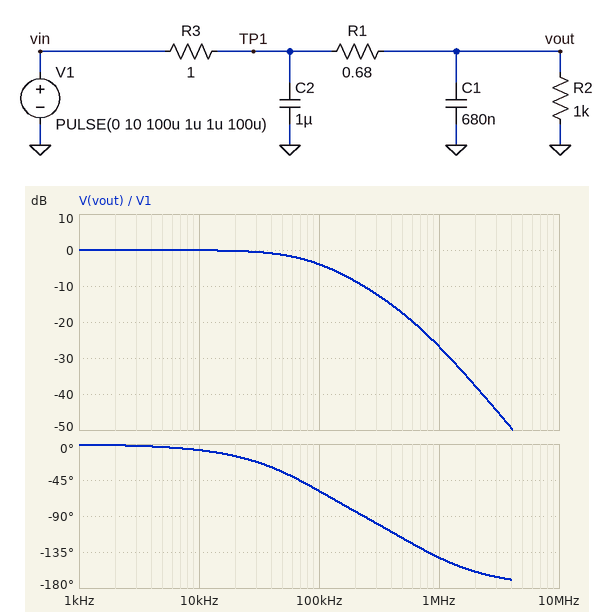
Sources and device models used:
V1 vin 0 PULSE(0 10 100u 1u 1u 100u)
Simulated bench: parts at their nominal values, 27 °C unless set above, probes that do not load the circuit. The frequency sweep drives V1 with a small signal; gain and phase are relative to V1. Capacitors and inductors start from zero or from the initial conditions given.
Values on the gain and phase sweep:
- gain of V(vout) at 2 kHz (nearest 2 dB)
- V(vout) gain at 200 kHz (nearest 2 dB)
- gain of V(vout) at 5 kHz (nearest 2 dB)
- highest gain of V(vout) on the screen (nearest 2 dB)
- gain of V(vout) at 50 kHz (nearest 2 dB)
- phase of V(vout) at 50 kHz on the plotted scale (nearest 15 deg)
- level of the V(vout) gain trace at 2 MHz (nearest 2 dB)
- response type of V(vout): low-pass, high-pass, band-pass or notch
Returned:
0 dB
-8 dB
0 dB
0 dB
-2 dB
-30 deg
-38 dB
low-pass
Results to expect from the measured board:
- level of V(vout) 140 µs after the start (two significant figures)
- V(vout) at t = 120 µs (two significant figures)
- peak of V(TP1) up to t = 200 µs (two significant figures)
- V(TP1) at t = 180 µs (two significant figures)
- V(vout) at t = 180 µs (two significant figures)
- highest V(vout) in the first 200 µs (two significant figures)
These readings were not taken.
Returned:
10 V
10 V
10 V
10 V
10 V
10 V
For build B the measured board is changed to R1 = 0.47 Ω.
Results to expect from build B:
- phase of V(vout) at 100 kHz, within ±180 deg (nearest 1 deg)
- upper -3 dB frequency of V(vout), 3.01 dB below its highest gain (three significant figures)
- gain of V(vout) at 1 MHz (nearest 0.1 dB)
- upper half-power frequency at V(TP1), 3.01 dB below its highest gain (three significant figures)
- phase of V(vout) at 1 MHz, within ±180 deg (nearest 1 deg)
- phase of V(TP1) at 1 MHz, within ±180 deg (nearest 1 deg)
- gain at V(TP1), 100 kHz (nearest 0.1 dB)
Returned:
-55 deg
86.6 kHz
-24.7 dB
89.3 kHz
-133 deg
-69 deg
-3.5 dB
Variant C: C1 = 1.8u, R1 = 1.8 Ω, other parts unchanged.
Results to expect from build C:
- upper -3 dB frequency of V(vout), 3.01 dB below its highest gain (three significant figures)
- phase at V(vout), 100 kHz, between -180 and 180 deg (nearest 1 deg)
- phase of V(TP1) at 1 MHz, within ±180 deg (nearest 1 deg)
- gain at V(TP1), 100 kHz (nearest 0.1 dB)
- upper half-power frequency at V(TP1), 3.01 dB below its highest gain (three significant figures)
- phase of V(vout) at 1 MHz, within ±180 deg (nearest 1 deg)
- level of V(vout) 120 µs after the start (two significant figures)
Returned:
29.0 kHz
-94 deg
-76 deg
-4.5 dB
50.4 kHz
-163 deg
9.7 V
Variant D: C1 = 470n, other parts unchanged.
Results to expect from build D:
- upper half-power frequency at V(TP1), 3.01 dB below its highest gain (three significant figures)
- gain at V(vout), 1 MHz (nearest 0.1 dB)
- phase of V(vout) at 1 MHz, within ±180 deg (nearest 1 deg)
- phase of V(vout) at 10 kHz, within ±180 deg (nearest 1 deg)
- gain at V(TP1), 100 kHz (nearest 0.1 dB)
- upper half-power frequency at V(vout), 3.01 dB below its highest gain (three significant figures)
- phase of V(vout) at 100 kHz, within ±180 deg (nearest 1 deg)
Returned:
103 kHz
-24.2 dB
-136 deg
-6 deg
-2.9 dB
98.8 kHz
-52 deg
